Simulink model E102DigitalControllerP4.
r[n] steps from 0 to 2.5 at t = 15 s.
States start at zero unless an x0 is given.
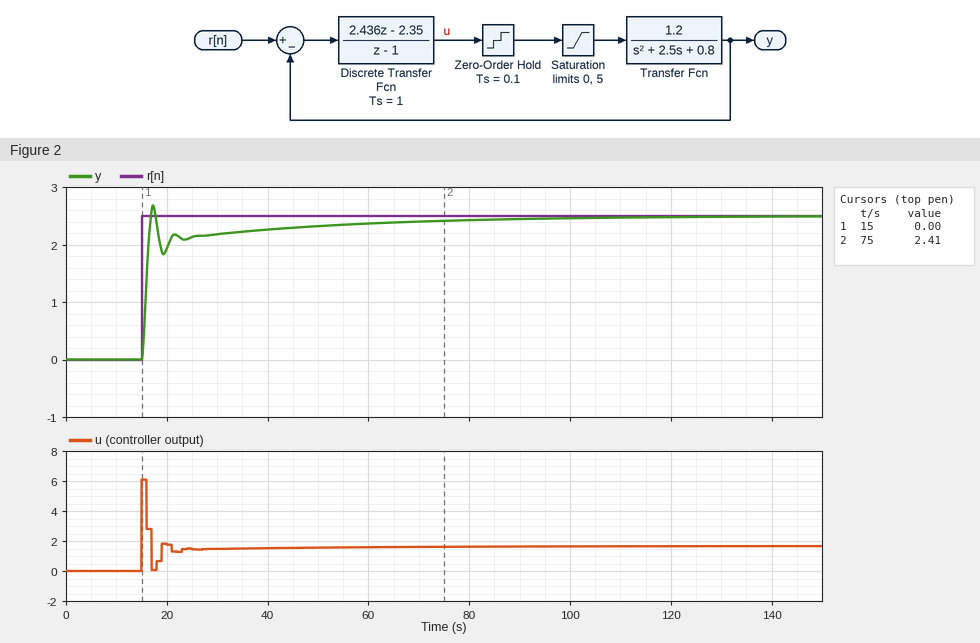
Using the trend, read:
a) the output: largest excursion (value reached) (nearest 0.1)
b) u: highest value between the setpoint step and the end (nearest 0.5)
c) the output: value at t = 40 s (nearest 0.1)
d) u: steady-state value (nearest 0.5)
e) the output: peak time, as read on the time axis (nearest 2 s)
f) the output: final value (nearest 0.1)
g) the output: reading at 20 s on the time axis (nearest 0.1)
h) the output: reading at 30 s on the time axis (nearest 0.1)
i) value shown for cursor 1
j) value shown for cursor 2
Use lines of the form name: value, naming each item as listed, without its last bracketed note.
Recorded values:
the output: largest excursion (value reached): 2.7
u: highest value between the setpoint step and the end: 6.0
the output: value at t = 40 s: 2.3
u: steady-state value: 1.5
the output: peak time, as read on the time axis: 18 s
the output: final value: 2.5
the output: reading at 20 s on the time axis: 1.9
the output: reading at 30 s on the time axis: 2.2
value shown for cursor 1: 0.00
value shown for cursor 2: 2.41
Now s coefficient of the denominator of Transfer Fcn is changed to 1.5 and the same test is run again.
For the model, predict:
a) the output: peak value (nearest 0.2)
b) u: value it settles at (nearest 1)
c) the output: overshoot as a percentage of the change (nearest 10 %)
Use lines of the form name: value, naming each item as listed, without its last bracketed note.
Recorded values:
the output: peak value: 3.4
u: value it settles at: 2
the output: overshoot as a percentage of the change: 30 %
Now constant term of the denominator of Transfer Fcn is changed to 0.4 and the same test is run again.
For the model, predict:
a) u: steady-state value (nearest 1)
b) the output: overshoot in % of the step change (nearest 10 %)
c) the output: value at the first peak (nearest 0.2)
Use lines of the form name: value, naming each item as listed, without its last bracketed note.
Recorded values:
u: steady-state value: 1
the output: overshoot in % of the step change: 20 %
the output: value at the first peak: 3.0
